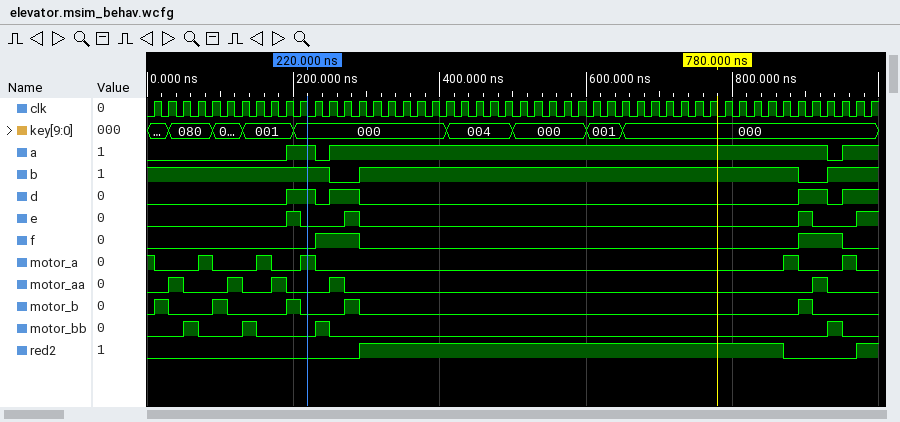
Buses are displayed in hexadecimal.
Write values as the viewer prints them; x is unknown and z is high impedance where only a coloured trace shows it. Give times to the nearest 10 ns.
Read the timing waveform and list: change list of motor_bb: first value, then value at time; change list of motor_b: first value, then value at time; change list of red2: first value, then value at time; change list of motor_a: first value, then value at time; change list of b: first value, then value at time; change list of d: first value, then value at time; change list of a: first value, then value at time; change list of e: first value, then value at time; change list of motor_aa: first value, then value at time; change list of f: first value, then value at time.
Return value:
0, 1 at 50 ns, 0 at 70 ns, 1 at 130 ns, 0 at 150 ns, 1 at 230 ns, 0 at 250 ns, 1 at 930 ns, 0 at 950 ns
0, 1 at 10 ns, 0 at 30 ns, 1 at 90 ns, 0 at 110 ns, 1 at 190 ns, 0 at 210 ns, 1 at 270 ns, 0 at 290 ns, 1 at 890 ns, 0 at 910 ns
0, 1 at 290 ns, 0 at 870 ns, 1 at 970 ns
1, 0 at 10 ns, 1 at 70 ns, 0 at 90 ns, 1 at 150 ns, 0 at 170 ns, 1 at 210 ns, 0 at 230 ns, 1 at 870 ns, 0 at 890 ns, 1 at 950 ns, 0 at 970 ns
1, 0 at 250 ns, 1 at 290 ns, 0 at 890 ns, 1 at 930 ns
0, 1 at 190 ns, 0 at 230 ns, 1 at 250 ns, 0 at 290 ns, 1 at 890 ns, 0 at 930 ns, 1 at 950 ns
0, 1 at 190 ns, 0 at 230 ns, 1 at 250 ns, 0 at 930 ns, 1 at 950 ns
0, 1 at 190 ns, 0 at 210 ns, 1 at 270 ns, 0 at 290 ns, 1 at 890 ns, 0 at 910 ns, 1 at 970 ns
0, 1 at 30 ns, 0 at 50 ns, 1 at 110 ns, 0 at 130 ns, 1 at 170 ns, 0 at 190 ns, 1 at 250 ns, 0 at 270 ns, 1 at 910 ns, 0 at 930 ns
0, 1 at 230 ns, 0 at 290 ns, 1 at 890 ns, 0 at 950 ns
